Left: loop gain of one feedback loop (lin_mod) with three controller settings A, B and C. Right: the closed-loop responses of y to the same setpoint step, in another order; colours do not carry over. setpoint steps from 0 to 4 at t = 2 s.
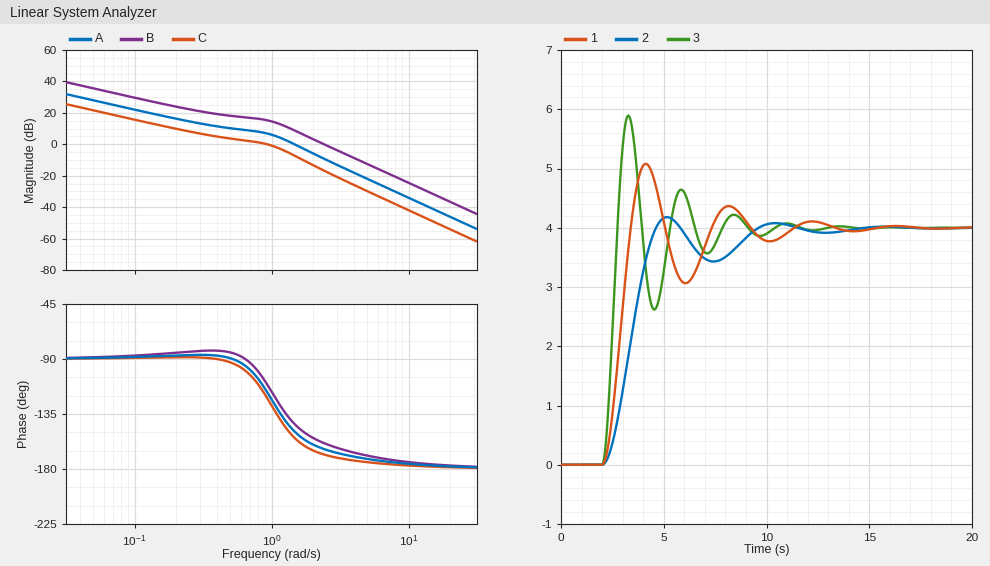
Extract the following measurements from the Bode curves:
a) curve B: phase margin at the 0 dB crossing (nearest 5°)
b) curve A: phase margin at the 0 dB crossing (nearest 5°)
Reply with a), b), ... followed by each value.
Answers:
a) 20°
b) 30°
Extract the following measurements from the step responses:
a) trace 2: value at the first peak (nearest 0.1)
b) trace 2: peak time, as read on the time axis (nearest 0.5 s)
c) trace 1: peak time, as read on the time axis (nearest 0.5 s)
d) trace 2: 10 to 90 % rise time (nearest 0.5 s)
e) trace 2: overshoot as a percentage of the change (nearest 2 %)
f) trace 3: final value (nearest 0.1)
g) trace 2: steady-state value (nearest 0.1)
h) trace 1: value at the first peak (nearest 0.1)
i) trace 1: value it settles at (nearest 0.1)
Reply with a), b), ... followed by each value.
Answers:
a) 4.2
b) 5.0 s
c) 4.0 s
d) 1.5 s
e) 4 %
f) 4.0
g) 4.0
h) 5.1
i) 4.0
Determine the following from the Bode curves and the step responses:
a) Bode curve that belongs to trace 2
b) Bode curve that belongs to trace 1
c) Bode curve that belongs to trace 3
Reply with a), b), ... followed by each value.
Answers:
a) C
b) A
c) B
